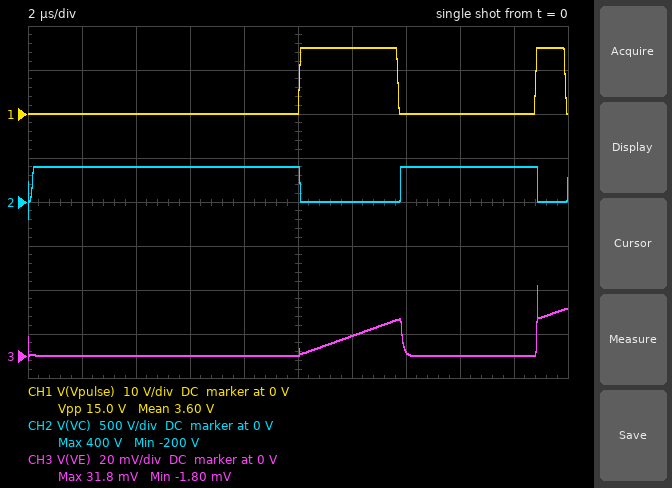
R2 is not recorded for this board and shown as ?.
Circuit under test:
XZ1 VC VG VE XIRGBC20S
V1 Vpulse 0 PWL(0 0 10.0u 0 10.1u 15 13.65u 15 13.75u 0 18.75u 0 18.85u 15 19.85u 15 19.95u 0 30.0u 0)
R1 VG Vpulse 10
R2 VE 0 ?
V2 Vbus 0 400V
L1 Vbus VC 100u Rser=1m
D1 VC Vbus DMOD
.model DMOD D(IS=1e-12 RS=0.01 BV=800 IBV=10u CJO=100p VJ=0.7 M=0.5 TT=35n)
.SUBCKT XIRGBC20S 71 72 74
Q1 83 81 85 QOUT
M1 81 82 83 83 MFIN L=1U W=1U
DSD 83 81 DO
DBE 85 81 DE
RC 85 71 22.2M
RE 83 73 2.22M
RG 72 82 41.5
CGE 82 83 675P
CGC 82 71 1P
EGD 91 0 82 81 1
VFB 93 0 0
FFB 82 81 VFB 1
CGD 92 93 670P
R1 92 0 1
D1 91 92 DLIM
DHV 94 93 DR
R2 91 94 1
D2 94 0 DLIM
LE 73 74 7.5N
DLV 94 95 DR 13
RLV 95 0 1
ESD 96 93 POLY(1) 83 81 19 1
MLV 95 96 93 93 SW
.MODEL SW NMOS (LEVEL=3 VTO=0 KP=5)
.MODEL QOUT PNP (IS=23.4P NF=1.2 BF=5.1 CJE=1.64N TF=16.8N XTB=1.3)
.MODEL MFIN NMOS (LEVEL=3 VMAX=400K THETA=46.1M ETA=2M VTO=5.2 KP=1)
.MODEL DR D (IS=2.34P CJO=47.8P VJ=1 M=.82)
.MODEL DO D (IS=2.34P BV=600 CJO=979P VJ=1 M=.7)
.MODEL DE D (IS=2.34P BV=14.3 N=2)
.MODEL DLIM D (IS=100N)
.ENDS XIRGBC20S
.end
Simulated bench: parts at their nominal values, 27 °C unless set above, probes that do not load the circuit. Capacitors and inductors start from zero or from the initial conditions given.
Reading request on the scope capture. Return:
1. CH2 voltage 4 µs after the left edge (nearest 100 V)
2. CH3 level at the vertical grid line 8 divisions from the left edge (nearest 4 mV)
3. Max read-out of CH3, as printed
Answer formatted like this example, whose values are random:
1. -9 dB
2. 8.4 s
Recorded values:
1. 400 V
2. 0 V
3. 31.8 mV
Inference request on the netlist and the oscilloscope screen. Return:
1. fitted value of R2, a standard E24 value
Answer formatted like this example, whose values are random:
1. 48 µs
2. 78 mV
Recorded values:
1. 1.1 mΩ
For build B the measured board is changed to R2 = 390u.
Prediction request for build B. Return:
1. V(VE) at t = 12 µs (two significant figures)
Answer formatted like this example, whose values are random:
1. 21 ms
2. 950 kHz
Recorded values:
1. 3.2 mV
